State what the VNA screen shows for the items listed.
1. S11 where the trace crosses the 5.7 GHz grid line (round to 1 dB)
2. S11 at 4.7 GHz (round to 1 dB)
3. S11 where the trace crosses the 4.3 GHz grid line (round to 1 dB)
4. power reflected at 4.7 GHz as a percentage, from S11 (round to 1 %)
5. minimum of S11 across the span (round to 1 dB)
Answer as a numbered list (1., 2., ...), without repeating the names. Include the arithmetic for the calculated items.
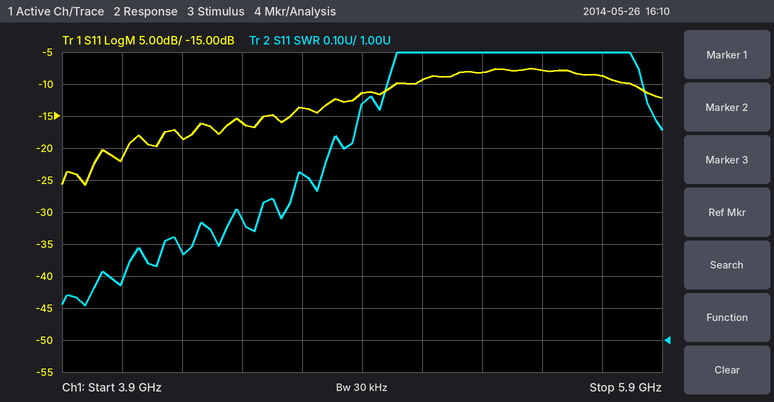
1. -9 dB
2. -14 dB
3. -18 dB
4. 10^(-14/10) ≈ 4 %
5. -26 dB
